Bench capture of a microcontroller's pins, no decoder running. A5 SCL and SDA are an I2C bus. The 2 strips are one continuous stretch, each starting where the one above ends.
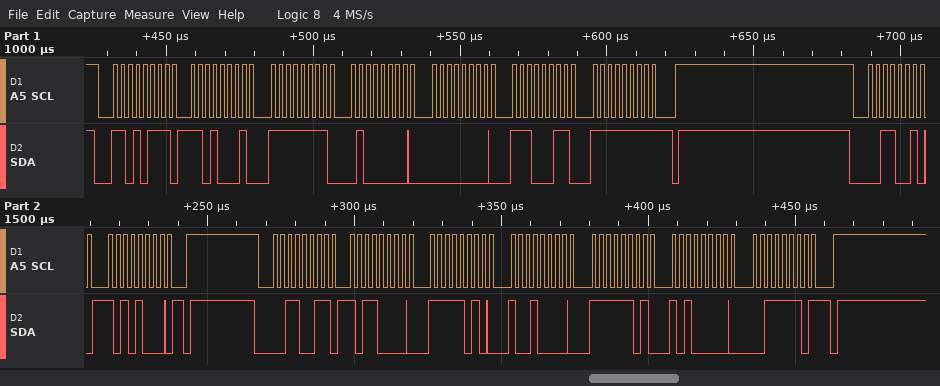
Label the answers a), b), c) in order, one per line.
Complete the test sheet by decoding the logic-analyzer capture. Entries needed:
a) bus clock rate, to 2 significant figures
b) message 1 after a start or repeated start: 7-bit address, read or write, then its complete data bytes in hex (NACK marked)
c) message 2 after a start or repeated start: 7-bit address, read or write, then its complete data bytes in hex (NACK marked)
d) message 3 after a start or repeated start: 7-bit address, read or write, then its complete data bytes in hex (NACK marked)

a) 400 kHz
b) 0x6B read: D1 FF 40 00 E3 FF NACK
c) 0x19 write: A8
d) 0x19 read: B0 FA 90 FD A0 3E NACK
